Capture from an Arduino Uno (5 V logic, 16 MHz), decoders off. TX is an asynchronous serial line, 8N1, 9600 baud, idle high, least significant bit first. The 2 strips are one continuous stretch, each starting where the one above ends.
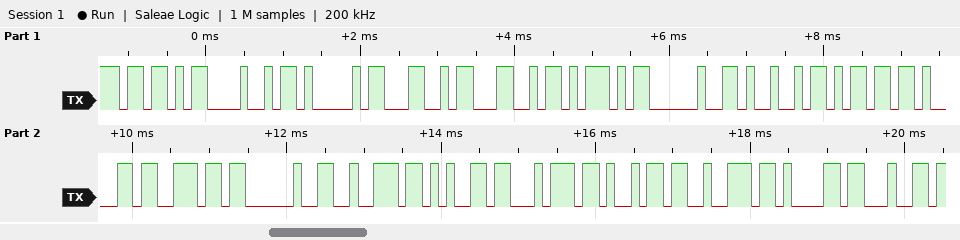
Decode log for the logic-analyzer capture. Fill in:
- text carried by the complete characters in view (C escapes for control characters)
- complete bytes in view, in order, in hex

"[HALL] Iman retirad"
0x5B 0x48 0x41 0x4C 0x4C 0x5D 0x20 0x49 0x6D 0x61 0x6E 0x20 0x72 0x65 0x74 0x69 0x72 0x61 0x64
